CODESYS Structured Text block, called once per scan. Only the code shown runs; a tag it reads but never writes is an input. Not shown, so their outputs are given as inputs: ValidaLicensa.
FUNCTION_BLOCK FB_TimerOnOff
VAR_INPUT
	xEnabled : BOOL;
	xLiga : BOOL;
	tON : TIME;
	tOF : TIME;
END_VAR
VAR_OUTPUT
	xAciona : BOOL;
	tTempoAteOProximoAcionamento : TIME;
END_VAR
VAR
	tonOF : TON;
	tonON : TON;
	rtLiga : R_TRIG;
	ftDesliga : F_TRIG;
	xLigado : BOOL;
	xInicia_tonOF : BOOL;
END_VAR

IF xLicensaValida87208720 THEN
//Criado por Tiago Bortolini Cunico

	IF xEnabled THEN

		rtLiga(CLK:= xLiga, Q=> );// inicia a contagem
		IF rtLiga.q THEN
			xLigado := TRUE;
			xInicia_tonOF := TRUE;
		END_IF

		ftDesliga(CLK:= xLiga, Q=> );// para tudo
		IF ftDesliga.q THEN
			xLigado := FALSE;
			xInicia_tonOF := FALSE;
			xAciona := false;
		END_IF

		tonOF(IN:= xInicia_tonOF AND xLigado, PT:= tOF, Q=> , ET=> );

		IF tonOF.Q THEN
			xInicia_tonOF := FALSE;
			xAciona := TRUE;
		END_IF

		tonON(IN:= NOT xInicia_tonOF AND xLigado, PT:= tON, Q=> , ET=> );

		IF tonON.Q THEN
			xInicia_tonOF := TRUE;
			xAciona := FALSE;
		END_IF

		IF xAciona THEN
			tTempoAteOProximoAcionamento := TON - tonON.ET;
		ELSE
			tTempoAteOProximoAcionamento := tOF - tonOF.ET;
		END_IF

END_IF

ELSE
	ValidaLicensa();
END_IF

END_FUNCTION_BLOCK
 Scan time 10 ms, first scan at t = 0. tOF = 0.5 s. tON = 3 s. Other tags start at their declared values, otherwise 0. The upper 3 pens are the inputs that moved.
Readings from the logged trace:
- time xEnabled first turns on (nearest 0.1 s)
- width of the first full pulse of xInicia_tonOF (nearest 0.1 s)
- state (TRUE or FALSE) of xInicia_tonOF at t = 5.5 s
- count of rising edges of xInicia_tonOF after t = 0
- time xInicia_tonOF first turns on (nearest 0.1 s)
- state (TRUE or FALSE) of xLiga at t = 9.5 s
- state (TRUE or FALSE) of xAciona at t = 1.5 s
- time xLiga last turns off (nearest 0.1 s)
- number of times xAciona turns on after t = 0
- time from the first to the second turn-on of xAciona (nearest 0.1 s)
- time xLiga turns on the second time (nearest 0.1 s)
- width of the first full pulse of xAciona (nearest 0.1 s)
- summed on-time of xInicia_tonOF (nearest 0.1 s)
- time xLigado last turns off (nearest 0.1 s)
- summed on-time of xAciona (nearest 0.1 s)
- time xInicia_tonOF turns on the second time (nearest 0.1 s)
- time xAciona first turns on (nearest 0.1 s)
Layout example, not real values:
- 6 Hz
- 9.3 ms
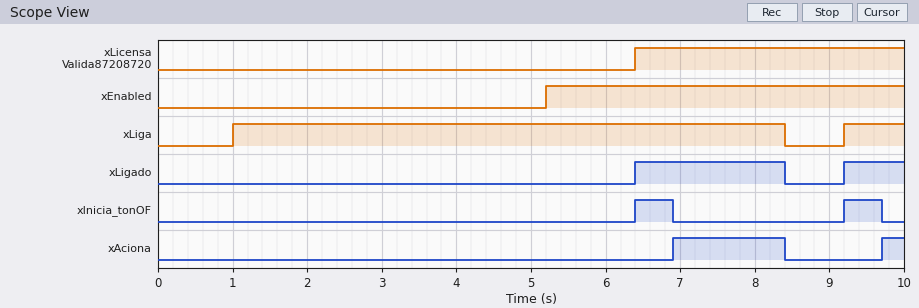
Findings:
- 5.2 s
- 0.5 s
- FALSE
- 2
- 6.4 s
- TRUE
- FALSE
- 8.4 s
- 2
- 2.8 s
- 9.2 s
- 1.5 s
- 1.0 s
- 8.4 s
- 1.8 s
- 9.2 s
- 6.9 s
